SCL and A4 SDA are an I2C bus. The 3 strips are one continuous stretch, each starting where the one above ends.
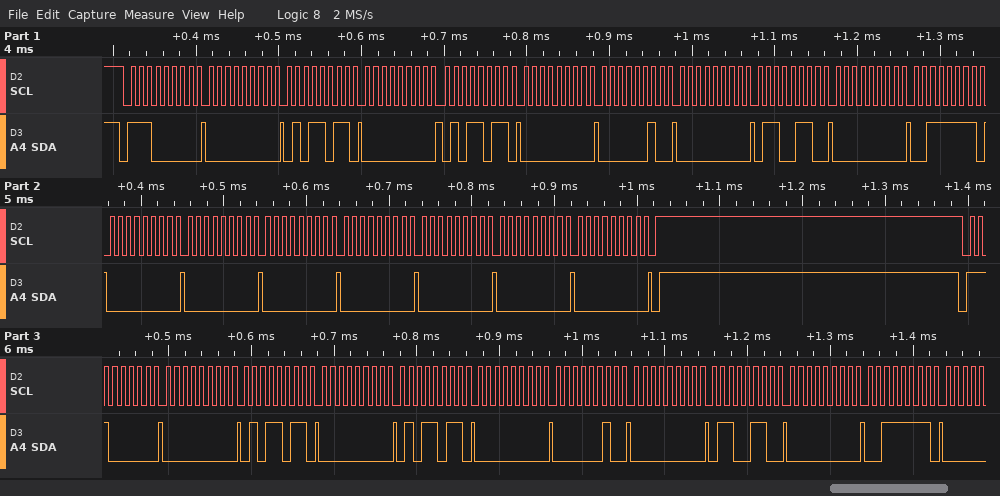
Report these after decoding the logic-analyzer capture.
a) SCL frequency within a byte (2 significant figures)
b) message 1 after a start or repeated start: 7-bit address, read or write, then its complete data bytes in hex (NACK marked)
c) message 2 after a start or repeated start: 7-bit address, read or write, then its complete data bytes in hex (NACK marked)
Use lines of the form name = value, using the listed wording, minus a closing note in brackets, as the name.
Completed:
SCL frequency within a byte = 100 kHz
message 1 after a start or repeated start: 7-bit address, read or write, then its complete data bytes in hex = 0x70 write: 00 5B 00 5B 00 02 00 66 00 3F 00 00 00 00 00 00 00
message 2 after a start or repeated start: 7-bit address, read or write, then its complete data bytes in hex = 0x70 write: 00 5B 00 5B 00 02 00 66 00 3F
